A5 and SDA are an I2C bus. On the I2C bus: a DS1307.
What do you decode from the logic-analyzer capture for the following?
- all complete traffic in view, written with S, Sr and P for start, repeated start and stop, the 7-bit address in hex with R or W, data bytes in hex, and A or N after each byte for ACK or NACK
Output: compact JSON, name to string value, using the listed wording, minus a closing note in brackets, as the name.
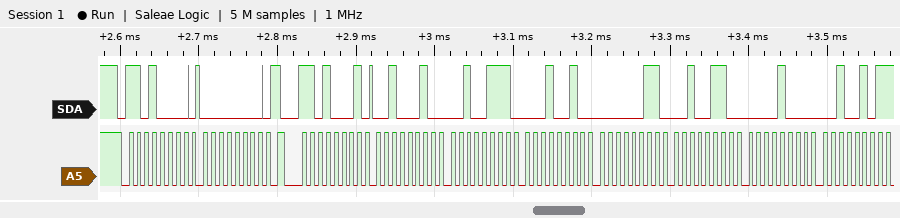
{"all complete traffic in view, written with S, Sr and P for start, repeated start and stop, the 7-bit address in hex with R or W, data bytes in hex, and A or N after each byte for ACK or NACK": "S 68W A 00 A Sr 68R A 22 A 27 A 12 A 03 A 26 A 08 A 25 N"}
